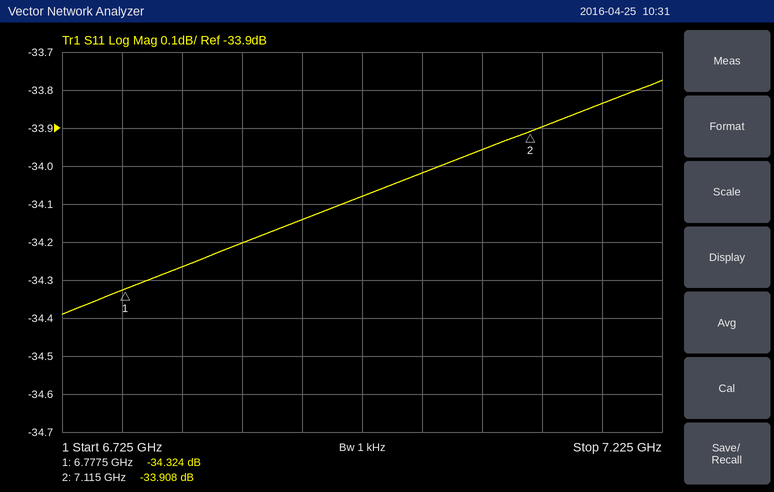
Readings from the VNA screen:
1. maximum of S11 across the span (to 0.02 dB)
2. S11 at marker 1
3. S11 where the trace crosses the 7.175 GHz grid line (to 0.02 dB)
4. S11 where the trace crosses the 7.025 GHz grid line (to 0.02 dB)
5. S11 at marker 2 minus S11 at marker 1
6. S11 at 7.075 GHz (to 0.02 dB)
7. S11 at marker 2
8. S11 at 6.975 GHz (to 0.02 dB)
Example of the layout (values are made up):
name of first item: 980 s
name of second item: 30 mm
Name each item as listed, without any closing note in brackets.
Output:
maximum of S11 across the span: -33.78 dB
S11 at marker 1: -34.324 dB
S11 where the trace crosses the 7.175 GHz grid line: -33.84 dB
S11 where the trace crosses the 7.025 GHz grid line: -34.02 dB
S11 at marker 2 minus S11 at marker 1: 0.416 dB
S11 at 7.075 GHz: -33.96 dB
S11 at marker 2: -33.908 dB
S11 at 6.975 GHz: -34.08 dB
